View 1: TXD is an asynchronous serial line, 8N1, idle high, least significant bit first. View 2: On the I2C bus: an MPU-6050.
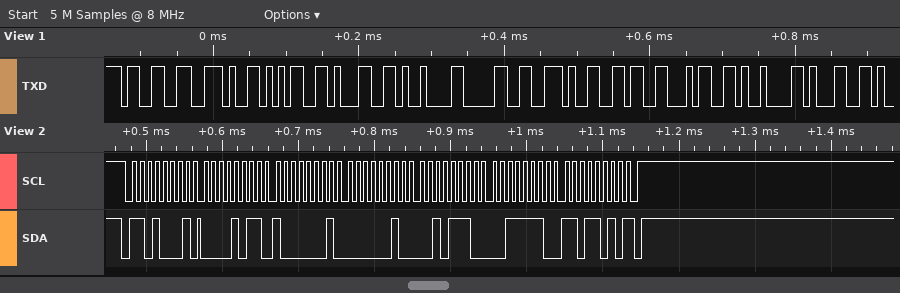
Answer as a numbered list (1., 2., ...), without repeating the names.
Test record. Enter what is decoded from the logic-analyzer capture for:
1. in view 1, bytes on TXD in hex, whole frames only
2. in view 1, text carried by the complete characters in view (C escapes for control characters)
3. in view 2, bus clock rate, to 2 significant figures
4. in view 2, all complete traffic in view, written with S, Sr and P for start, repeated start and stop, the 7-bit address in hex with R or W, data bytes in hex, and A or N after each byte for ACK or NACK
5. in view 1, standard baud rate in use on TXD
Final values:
1. 0x33 0x2E 0x35 0x31 0x09 0x30 0x2E 0x36 0x34 0x09 0x31
2. "3.51\t0.64\t1"
3. 100 kHz
4. S 68R A 0B A 81 A 02 A 2E A 3E A DA N P
5. 115200 baud
